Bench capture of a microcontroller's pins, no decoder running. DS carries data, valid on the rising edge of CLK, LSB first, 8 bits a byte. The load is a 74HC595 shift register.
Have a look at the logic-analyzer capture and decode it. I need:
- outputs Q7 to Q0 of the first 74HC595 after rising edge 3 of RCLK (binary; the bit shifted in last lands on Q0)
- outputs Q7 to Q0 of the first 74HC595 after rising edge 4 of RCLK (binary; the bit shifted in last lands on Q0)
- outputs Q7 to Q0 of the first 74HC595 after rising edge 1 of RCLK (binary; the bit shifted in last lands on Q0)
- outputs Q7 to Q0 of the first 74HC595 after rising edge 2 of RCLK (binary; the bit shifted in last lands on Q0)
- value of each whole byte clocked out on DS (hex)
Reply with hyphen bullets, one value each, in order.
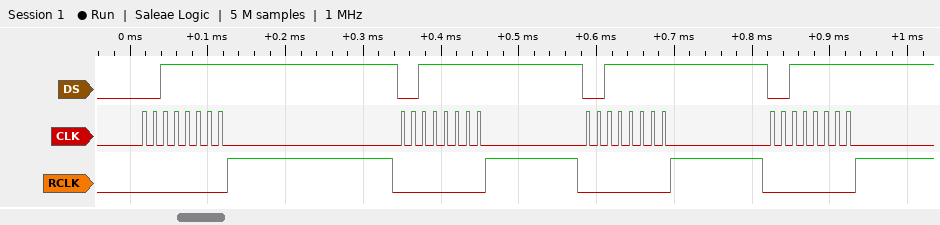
- 00111111
- 00111111
- 00111111
- 00111111
- 0xFC 0xFC 0xFC 0xFC
